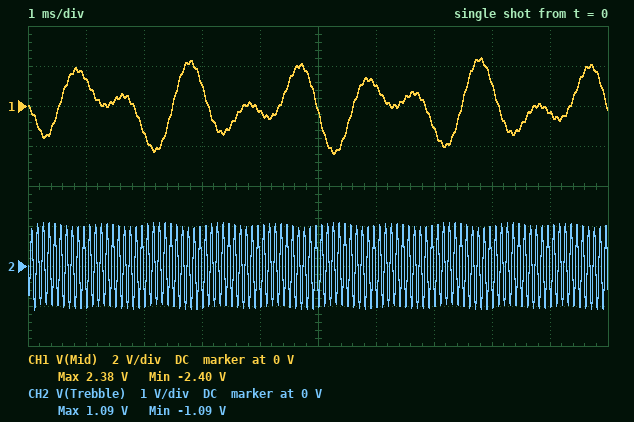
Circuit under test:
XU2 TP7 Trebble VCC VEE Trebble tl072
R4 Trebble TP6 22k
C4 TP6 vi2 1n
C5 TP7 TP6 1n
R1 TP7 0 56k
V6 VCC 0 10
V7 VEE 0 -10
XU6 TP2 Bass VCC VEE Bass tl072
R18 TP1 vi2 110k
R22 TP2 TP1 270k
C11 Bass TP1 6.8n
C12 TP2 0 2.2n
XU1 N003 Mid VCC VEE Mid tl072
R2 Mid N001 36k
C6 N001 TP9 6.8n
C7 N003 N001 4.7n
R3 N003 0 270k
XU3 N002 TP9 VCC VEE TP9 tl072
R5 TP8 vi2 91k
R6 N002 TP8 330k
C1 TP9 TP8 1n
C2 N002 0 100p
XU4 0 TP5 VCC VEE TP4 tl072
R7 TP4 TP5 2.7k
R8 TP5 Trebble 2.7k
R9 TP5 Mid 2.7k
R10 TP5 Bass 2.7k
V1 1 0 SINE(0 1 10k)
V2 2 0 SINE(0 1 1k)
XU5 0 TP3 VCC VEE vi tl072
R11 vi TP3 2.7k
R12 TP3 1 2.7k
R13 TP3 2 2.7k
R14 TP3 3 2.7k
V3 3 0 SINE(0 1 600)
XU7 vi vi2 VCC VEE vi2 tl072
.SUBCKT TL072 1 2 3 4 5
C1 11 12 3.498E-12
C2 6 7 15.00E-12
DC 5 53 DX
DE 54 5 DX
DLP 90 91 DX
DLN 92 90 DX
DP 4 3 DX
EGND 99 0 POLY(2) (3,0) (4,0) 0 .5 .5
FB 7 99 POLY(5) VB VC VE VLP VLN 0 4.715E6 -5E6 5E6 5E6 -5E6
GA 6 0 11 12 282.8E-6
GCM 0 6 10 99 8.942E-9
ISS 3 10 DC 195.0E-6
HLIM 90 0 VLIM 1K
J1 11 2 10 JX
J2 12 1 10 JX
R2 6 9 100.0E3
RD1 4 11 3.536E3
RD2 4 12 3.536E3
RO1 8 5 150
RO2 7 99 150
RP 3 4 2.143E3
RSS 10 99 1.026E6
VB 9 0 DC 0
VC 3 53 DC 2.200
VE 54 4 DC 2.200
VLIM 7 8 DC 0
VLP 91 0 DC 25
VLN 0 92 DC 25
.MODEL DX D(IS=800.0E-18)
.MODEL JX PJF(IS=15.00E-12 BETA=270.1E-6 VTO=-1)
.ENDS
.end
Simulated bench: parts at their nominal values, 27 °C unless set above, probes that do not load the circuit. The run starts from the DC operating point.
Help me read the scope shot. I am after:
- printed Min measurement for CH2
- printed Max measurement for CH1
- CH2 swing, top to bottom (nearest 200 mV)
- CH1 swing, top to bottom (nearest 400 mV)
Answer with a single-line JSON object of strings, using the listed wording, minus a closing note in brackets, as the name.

{"printed Min measurement for CH2": "-1.09 V", "printed Max measurement for CH1": "2.38 V", "CH2 swing, top to bottom": "2.2 V", "CH1 swing, top to bottom": "4.8 V"}
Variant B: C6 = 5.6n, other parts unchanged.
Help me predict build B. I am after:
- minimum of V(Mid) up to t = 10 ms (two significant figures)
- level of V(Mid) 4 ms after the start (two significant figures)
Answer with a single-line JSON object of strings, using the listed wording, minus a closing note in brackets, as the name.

{"minimum of V(Mid) up to t = 10 ms": "-2.5 V", "level of V(Mid) 4 ms after the start": "-250 mV"}
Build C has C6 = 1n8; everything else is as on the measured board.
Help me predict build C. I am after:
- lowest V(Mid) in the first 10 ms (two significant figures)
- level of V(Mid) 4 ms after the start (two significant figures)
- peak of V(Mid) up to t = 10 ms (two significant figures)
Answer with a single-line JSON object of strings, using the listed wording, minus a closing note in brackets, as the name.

{"lowest V(Mid) in the first 10 ms": "-2.7 V", "level of V(Mid) 4 ms after the start": "400 mV", "peak of V(Mid) up to t = 10 ms": "2.6 V"}
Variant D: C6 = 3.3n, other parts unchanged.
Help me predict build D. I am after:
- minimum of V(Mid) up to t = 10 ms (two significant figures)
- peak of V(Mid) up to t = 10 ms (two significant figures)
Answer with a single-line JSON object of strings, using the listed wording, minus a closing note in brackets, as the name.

{"minimum of V(Mid) up to t = 10 ms": "-2.7 V", "peak of V(Mid) up to t = 10 ms": "2.8 V"}
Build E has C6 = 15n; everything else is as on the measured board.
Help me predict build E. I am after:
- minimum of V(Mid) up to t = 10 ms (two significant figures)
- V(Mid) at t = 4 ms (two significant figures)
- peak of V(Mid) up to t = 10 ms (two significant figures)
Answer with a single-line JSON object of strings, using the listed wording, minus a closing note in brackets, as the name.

{"minimum of V(Mid) up to t = 10 ms": "-2.2 V", "V(Mid) at t = 4 ms": "-430 mV", "peak of V(Mid) up to t = 10 ms": "2.2 V"}
